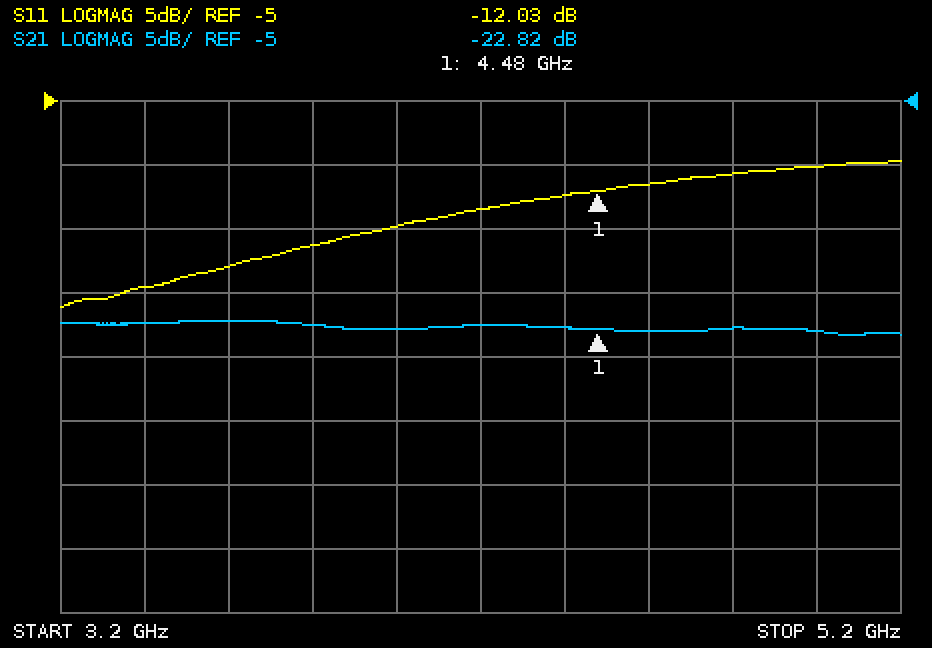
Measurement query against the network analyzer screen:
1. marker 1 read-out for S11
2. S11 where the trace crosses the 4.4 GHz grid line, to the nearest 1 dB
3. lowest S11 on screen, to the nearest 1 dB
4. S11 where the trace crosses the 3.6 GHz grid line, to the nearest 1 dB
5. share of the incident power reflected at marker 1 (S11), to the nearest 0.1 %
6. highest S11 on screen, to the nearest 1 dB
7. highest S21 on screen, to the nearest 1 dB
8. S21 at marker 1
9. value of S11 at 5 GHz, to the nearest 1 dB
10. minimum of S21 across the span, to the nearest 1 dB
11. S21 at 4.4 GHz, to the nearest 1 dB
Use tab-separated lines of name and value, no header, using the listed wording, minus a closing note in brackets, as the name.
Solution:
marker 1 read-out for S11	-12.03 dB
S11 where the trace crosses the 4.4 GHz grid line, to the nearest 1 dB	-12 dB
lowest S11 on screen, to the nearest 1 dB	-21 dB
S11 where the trace crosses the 3.6 GHz grid line, to the nearest 1 dB	-18 dB
share of the incident power reflected at marker 1 (S11), to the nearest 0.1 %	6.3 %
highest S11 on screen, to the nearest 1 dB	-10 dB
highest S21 on screen, to the nearest 1 dB	-22 dB
S21 at marker 1	-22.82 dB
value of S11 at 5 GHz, to the nearest 1 dB	-10 dB
minimum of S21 across the span, to the nearest 1 dB	-23 dB
S21 at 4.4 GHz, to the nearest 1 dB	-23 dB
